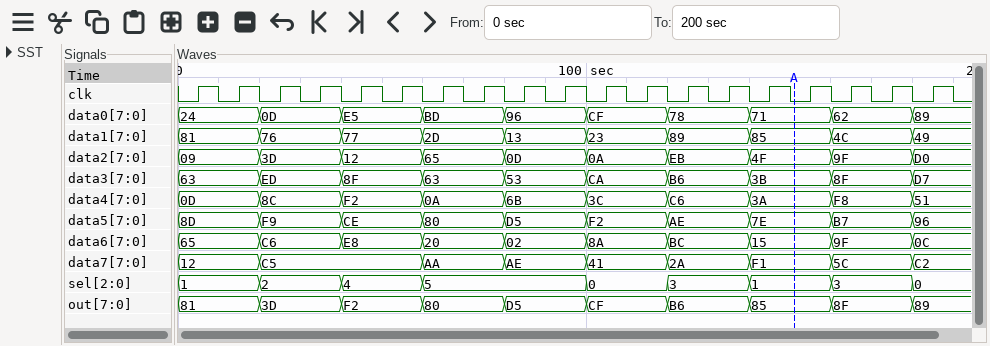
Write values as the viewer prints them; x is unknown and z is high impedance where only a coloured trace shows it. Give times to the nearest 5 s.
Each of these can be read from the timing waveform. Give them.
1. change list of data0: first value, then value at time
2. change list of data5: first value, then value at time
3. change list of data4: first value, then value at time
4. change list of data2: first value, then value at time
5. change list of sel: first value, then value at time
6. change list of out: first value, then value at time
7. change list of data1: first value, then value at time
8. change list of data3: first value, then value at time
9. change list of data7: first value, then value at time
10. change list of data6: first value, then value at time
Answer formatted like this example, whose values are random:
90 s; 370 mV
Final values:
24, 0D at 20 s, E5 at 40 s, BD at 60 s, 96 at 80 s, CF at 100 s, 78 at 120 s, 71 at 140 s, 62 at 160 s, 89 at 180 s; 8D, F9 at 20 s, CE at 40 s, 80 at 60 s, D5 at 80 s, F2 at 100 s, AE at 120 s, 7E at 140 s, B7 at 160 s, 96 at 180 s; 0D, 8C at 20 s, F2 at 40 s, 0A at 60 s, 6B at 80 s, 3C at 100 s, C6 at 120 s, 3A at 140 s, F8 at 160 s, 51 at 180 s; 09, 3D at 20 s, 12 at 40 s, 65 at 60 s, 0D at 80 s, 0A at 100 s, EB at 120 s, 4F at 140 s, 9F at 160 s, D0 at 180 s; 1, 2 at 20 s, 4 at 40 s, 5 at 60 s, 0 at 100 s, 3 at 120 s, 1 at 140 s, 3 at 160 s, 0 at 180 s; 81, 3D at 20 s, F2 at 40 s, 80 at 60 s, D5 at 80 s, CF at 100 s, B6 at 120 s, 85 at 140 s, 8F at 160 s, 89 at 180 s; 81, 76 at 20 s, 77 at 40 s, 2D at 60 s, 13 at 80 s, 23 at 100 s, 89 at 120 s, 85 at 140 s, 4C at 160 s, 49 at 180 s; 63, ED at 20 s, 8F at 40 s, 63 at 60 s, 53 at 80 s, CA at 100 s, B6 at 120 s, 3B at 140 s, 8F at 160 s, D7 at 180 s; 12, C5 at 20 s, AA at 60 s, AE at 80 s, 41 at 100 s, 2A at 120 s, F1 at 140 s, 5C at 160 s, C2 at 180 s; 65, C6 at 20 s, E8 at 40 s, 20 at 60 s, 02 at 80 s, 8A at 100 s, BC at 120 s, 15 at 140 s, 9F at 160 s, 0C at 180 s
